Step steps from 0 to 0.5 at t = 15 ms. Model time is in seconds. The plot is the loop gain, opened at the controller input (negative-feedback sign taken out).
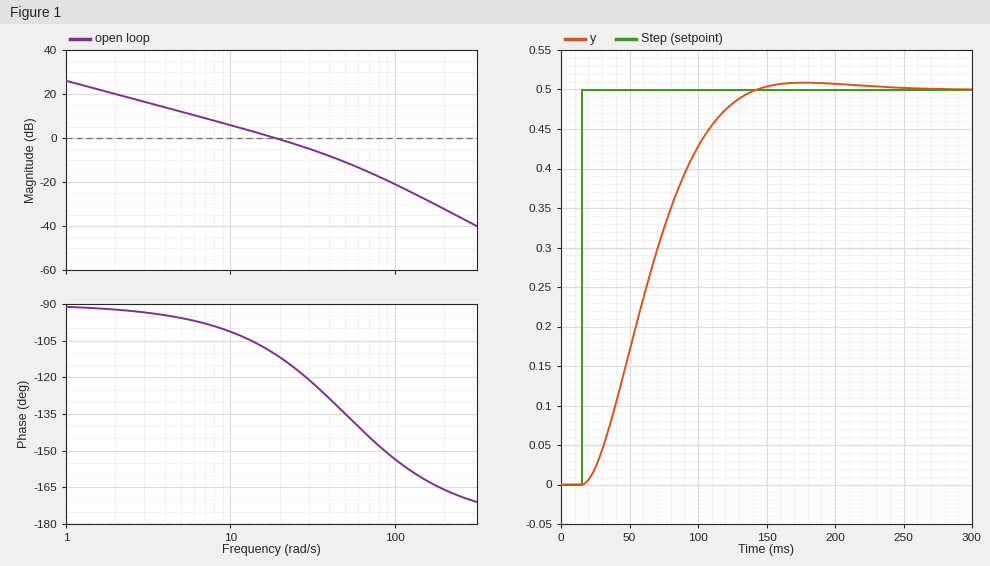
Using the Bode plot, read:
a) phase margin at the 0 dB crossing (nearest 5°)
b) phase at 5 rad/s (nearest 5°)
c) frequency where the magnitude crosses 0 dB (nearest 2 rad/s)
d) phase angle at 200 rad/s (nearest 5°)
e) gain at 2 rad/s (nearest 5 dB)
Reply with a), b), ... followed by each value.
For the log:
a) 70°
b) -95°
c) 18 rad/s
d) -165°
e) 20 dB
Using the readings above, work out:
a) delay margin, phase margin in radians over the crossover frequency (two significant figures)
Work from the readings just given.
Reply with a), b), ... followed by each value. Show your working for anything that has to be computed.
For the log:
a) 70 × π / 180 / 18 = 0.068 s
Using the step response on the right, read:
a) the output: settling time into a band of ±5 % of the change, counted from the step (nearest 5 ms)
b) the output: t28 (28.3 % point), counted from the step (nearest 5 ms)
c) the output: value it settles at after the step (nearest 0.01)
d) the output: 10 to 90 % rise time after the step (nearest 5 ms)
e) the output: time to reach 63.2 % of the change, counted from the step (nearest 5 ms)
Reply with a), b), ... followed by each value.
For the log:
a) 105 ms
b) 30 ms
c) 0.50
d) 75 ms
e) 60 ms
